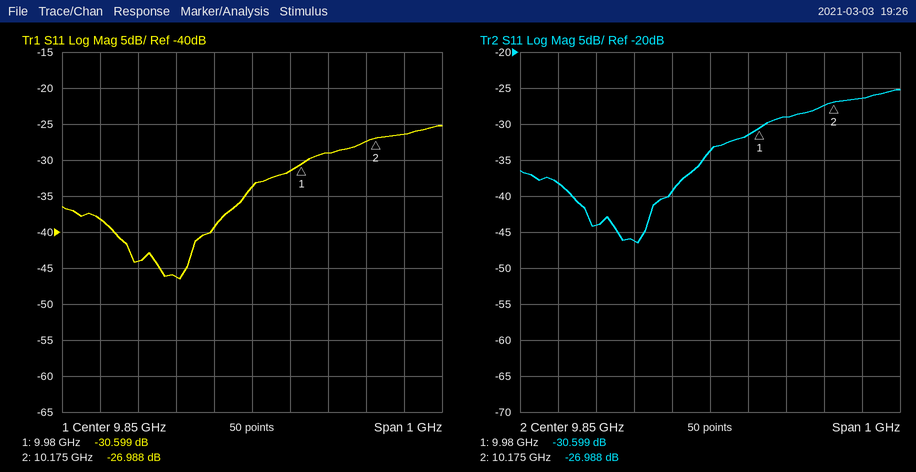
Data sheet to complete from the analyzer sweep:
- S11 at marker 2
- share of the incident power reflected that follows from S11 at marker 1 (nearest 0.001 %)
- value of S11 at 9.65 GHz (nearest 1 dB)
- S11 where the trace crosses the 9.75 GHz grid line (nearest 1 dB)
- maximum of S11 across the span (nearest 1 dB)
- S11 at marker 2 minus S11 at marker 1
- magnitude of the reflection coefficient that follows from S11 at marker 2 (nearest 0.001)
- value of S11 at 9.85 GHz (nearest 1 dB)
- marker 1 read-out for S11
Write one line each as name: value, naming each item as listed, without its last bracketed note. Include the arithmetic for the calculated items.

S11 at marker 2: -26.988 dB
share of the incident power reflected that follows from S11 at marker 1: 10^(-30.599/10) ≈ 0.087 %
value of S11 at 9.65 GHz: -46 dB
S11 where the trace crosses the 9.75 GHz grid line: -39 dB
maximum of S11 across the span: -25 dB
S11 at marker 2 minus S11 at marker 1: -26.988 − (-30.599) = 3.611 dB
magnitude of the reflection coefficient that follows from S11 at marker 2: 10^(-26.988/20) ≈ 0.045
value of S11 at 9.85 GHz: -34 dB
marker 1 read-out for S11: -30.599 dB
